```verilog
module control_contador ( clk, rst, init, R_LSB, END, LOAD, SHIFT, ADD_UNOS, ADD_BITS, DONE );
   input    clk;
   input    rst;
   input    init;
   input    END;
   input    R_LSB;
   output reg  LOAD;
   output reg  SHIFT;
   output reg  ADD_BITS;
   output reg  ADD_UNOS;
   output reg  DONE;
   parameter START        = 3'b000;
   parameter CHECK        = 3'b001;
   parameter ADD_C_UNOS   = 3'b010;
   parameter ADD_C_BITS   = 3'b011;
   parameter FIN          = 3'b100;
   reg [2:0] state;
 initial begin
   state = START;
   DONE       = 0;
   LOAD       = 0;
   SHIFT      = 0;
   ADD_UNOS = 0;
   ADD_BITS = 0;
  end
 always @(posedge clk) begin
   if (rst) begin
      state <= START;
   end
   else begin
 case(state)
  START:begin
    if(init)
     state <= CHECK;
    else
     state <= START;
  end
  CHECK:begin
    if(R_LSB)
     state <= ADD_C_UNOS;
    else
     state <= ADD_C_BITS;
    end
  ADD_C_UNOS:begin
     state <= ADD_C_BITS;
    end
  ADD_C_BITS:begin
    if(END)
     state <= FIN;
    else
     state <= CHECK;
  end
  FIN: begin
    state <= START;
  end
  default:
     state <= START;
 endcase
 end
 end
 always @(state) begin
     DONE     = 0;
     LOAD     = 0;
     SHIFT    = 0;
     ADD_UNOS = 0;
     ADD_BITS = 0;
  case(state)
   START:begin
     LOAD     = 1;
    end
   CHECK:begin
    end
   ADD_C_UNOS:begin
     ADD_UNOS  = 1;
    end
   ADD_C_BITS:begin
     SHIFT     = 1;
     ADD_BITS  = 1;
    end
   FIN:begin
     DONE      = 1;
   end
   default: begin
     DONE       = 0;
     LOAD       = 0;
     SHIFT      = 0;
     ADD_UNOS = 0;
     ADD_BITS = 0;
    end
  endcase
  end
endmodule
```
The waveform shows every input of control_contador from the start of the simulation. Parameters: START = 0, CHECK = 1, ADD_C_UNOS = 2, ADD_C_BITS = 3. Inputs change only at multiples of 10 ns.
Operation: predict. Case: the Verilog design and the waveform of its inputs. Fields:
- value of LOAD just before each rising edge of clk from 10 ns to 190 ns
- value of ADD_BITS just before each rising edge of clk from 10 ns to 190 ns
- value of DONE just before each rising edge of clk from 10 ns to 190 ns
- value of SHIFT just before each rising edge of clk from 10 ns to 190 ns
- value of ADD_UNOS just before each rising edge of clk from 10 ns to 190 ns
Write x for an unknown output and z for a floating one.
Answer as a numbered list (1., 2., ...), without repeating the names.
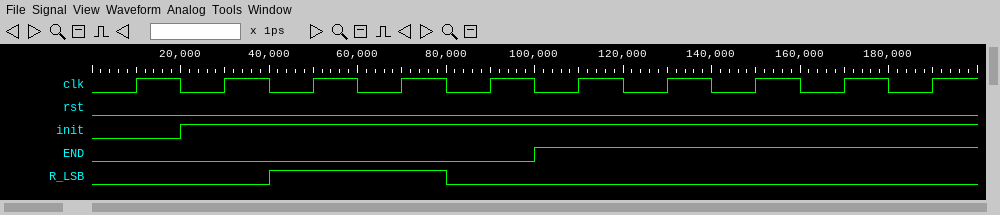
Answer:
1. 1 1 0 0 0 0 0 0 1 0
2. 0 0 0 0 1 0 1 0 0 0
3. 0 0 0 0 0 0 0 1 0 0
4. 0 0 0 0 1 0 1 0 0 0
5. 0 0 0 1 0 0 0 0 0 0
